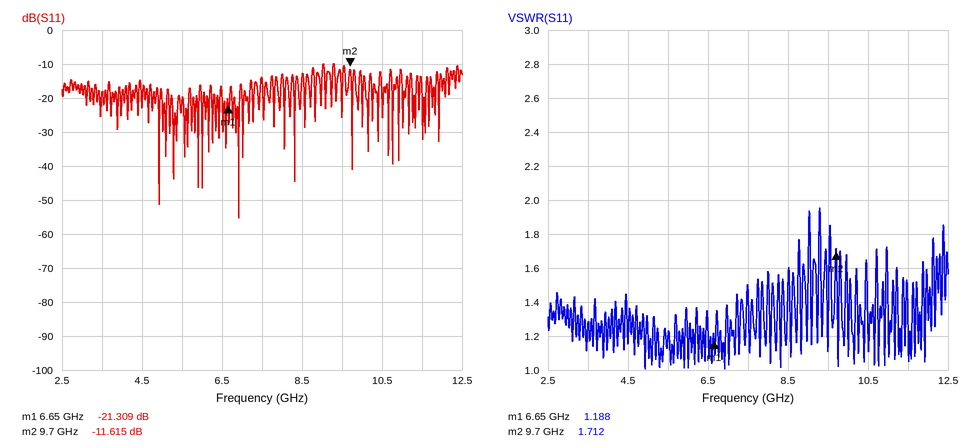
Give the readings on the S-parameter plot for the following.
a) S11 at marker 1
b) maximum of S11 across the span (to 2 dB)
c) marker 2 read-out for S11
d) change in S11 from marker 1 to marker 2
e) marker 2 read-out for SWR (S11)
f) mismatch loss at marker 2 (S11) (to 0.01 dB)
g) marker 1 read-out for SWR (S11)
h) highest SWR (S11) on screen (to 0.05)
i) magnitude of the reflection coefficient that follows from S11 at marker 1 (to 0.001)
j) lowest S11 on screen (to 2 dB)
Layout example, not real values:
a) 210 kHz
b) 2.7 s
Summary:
a) -21.309 dB
b) -10 dB
c) -11.615 dB
d) 9.694 dB
e) 1.712
f) 0.31 dB
g) 1.188
h) 1.95
i) 0.086
j) -56 dB
